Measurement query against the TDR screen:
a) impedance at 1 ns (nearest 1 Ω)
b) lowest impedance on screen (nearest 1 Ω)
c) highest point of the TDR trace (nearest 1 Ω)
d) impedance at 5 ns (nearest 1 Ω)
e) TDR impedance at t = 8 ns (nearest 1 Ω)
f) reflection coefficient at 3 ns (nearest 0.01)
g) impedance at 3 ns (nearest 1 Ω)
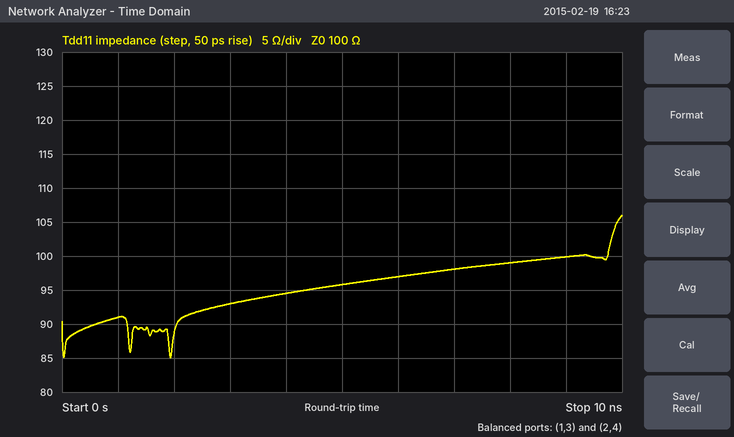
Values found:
91 Ω
85 Ω
106 Ω
96 Ω
99 Ω
-0.04
93 Ω
